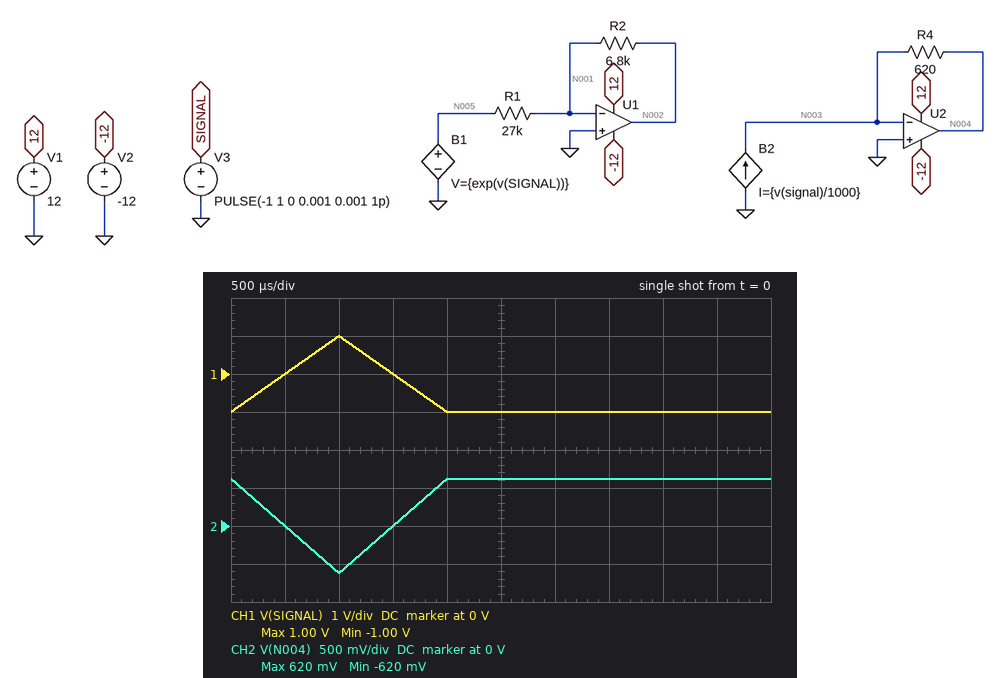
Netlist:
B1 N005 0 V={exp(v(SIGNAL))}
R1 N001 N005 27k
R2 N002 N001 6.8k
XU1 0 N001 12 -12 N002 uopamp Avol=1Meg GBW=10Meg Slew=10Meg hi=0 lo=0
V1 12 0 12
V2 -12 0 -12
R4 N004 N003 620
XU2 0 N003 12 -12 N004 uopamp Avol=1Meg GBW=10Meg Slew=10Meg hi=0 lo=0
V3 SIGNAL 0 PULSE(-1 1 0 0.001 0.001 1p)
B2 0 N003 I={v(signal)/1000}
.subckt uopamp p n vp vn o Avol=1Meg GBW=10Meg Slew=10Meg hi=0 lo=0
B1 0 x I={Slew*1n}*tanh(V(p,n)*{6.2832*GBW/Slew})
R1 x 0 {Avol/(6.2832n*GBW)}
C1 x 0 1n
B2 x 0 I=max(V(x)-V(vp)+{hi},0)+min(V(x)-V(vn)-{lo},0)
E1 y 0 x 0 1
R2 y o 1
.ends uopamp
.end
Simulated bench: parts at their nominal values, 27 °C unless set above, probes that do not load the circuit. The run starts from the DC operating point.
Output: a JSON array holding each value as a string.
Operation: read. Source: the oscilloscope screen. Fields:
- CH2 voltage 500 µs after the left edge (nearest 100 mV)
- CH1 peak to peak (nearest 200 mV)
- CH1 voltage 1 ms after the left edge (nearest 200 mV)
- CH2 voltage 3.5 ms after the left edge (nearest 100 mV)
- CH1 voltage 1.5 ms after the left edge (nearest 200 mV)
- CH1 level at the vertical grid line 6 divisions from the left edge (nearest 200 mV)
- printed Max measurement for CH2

["0 V", "2.0 V", "1.0 V", "600 mV", "0 V", "-1.0 V", "620 mV"]
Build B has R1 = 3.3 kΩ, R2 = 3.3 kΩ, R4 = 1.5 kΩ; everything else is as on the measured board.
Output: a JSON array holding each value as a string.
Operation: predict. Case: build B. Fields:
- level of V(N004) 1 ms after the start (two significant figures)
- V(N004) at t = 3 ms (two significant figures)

["-1.5 V", "1.5 V"]
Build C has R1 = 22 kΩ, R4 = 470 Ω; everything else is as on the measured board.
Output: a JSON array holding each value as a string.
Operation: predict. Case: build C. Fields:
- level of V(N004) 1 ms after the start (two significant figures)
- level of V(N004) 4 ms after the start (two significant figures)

["-470 mV", "470 mV"]
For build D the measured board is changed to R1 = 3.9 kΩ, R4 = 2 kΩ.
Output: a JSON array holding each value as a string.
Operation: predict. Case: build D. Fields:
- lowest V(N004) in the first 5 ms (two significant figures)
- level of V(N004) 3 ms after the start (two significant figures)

["-2.0 V", "2.0 V"]
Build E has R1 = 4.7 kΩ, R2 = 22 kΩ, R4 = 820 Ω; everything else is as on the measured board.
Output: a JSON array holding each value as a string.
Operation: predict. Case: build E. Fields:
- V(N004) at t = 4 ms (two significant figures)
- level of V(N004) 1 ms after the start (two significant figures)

["820 mV", "-820 mV"]
